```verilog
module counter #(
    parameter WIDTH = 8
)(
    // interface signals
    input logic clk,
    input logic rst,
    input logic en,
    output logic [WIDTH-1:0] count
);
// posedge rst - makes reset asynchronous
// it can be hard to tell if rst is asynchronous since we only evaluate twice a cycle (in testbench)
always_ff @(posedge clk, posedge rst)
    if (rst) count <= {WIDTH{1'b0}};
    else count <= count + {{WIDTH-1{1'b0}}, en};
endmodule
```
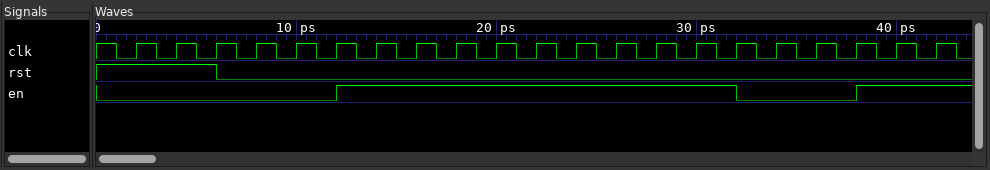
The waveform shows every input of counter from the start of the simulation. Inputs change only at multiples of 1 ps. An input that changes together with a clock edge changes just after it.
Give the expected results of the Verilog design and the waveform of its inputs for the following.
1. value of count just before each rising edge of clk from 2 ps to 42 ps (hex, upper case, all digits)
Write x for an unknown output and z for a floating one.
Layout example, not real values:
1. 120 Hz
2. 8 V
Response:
1. 00, 00, 00, 00, 00, 00, 00, 01, 02, 03, 04, 05, 06, 07, 08, 09, 0A, 0A, 0A, 0A, 0B
